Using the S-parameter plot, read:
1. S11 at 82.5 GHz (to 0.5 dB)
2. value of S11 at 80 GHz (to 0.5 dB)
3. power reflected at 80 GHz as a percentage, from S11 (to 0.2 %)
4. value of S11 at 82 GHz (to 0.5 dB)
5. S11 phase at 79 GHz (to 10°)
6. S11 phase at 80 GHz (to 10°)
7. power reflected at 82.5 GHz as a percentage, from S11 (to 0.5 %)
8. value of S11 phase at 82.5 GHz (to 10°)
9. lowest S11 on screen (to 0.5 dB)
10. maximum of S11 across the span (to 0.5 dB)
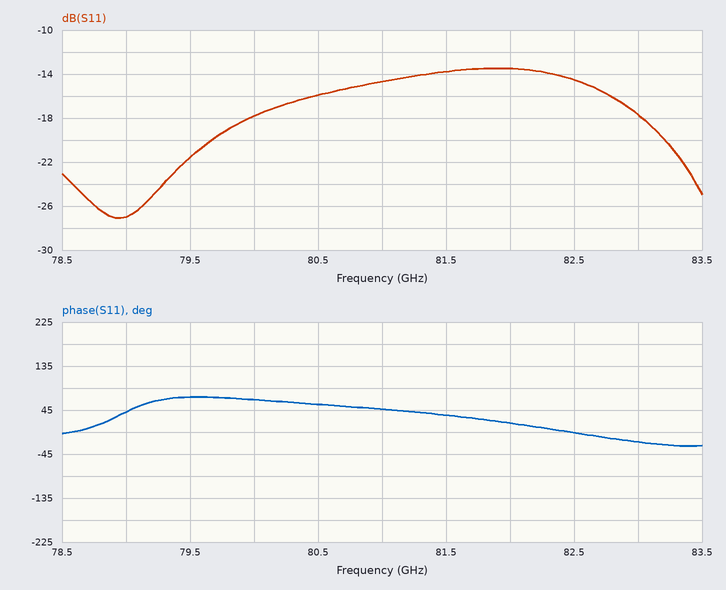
-14.5 dB
-18.0 dB
1.6 %
-13.5 dB
40°
70°
3.5 %
0°
-27.0 dB
-13.5 dB
